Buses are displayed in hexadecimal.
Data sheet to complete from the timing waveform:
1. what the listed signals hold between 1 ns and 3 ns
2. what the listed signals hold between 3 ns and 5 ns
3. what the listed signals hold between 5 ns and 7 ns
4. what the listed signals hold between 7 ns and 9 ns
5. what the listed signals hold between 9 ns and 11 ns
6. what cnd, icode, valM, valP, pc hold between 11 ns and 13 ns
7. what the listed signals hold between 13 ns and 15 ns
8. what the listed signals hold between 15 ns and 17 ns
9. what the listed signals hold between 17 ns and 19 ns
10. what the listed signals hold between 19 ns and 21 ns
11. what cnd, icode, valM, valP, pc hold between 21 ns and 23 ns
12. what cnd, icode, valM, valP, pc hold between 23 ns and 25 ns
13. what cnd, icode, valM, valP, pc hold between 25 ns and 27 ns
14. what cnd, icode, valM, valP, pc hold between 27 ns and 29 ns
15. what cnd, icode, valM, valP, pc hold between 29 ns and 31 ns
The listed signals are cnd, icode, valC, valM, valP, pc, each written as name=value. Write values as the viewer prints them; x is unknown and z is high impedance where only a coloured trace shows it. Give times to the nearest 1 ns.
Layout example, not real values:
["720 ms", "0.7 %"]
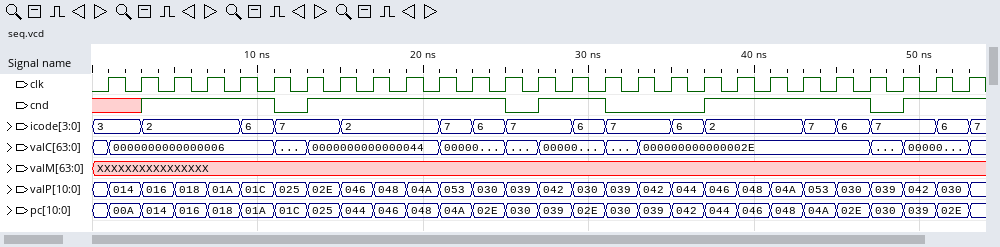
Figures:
["cnd=x, icode=3, valC=0000000000000006, valM=XXXXXXXXXXXXXXXX, valP=014, pc=00A", "cnd=1, icode=2, valC=0000000000000006, valM=XXXXXXXXXXXXXXXX, valP=016, pc=014", "cnd=1, icode=2, valC=0000000000000006, valM=XXXXXXXXXXXXXXXX, valP=018, pc=016", "cnd=1, icode=2, valC=0000000000000006, valM=XXXXXXXXXXXXXXXX, valP=01A, pc=018", "cnd=1, icode=6, valC=0000000000000006, valM=XXXXXXXXXXXXXXXX, valP=01C, pc=01A", "cnd=0, icode=7, valM=XXXXXXXXXXXXXXXX, valP=025, pc=01C", "cnd=1, icode=7, valC=0000000000000044, valM=XXXXXXXXXXXXXXXX, valP=02E, pc=025", "cnd=1, icode=2, valC=0000000000000044, valM=XXXXXXXXXXXXXXXX, valP=046, pc=044", "cnd=1, icode=2, valC=0000000000000044, valM=XXXXXXXXXXXXXXXX, valP=048, pc=046", "cnd=1, icode=2, valC=0000000000000044, valM=XXXXXXXXXXXXXXXX, valP=04A, pc=048", "cnd=1, icode=7, valM=XXXXXXXXXXXXXXXX, valP=053, pc=04A", "cnd=1, icode=6, valM=XXXXXXXXXXXXXXXX, valP=030, pc=02E", "cnd=0, icode=7, valM=XXXXXXXXXXXXXXXX, valP=039, pc=030", "cnd=1, icode=7, valM=XXXXXXXXXXXXXXXX, valP=042, pc=039", "cnd=1, icode=6, valM=XXXXXXXXXXXXXXXX, valP=030, pc=02E"]
